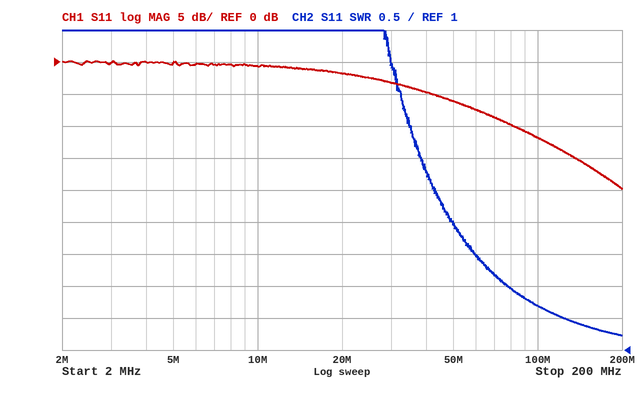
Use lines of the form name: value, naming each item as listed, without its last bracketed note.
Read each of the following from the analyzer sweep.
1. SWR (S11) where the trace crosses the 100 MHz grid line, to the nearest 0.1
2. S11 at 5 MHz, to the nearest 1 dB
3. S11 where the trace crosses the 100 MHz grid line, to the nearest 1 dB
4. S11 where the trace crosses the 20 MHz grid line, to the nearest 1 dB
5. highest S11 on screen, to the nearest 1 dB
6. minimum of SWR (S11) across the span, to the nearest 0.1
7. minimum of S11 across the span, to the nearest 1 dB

SWR (S11) where the trace crosses the 100 MHz grid line, to the nearest 0.1: 1.7
S11 at 5 MHz, to the nearest 1 dB: 0 dB
S11 where the trace crosses the 100 MHz grid line, to the nearest 1 dB: -12 dB
S11 where the trace crosses the 20 MHz grid line, to the nearest 1 dB: -2 dB
highest S11 on screen, to the nearest 1 dB: 0 dB
minimum of SWR (S11) across the span, to the nearest 0.1: 1.2
minimum of S11 across the span, to the nearest 1 dB: -20 dB
